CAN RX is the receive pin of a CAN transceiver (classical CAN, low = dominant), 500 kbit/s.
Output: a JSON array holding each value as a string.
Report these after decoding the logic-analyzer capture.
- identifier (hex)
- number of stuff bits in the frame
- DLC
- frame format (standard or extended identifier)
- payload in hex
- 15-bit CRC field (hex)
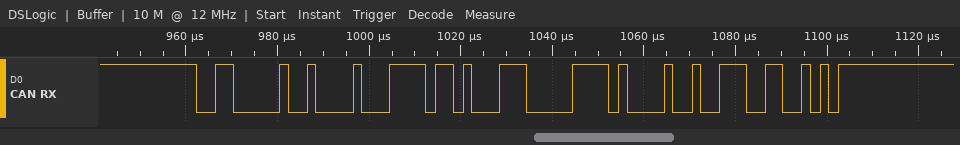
["0x301", "2", "4", "standard", "7B 47 07 42", "0x2732"]
